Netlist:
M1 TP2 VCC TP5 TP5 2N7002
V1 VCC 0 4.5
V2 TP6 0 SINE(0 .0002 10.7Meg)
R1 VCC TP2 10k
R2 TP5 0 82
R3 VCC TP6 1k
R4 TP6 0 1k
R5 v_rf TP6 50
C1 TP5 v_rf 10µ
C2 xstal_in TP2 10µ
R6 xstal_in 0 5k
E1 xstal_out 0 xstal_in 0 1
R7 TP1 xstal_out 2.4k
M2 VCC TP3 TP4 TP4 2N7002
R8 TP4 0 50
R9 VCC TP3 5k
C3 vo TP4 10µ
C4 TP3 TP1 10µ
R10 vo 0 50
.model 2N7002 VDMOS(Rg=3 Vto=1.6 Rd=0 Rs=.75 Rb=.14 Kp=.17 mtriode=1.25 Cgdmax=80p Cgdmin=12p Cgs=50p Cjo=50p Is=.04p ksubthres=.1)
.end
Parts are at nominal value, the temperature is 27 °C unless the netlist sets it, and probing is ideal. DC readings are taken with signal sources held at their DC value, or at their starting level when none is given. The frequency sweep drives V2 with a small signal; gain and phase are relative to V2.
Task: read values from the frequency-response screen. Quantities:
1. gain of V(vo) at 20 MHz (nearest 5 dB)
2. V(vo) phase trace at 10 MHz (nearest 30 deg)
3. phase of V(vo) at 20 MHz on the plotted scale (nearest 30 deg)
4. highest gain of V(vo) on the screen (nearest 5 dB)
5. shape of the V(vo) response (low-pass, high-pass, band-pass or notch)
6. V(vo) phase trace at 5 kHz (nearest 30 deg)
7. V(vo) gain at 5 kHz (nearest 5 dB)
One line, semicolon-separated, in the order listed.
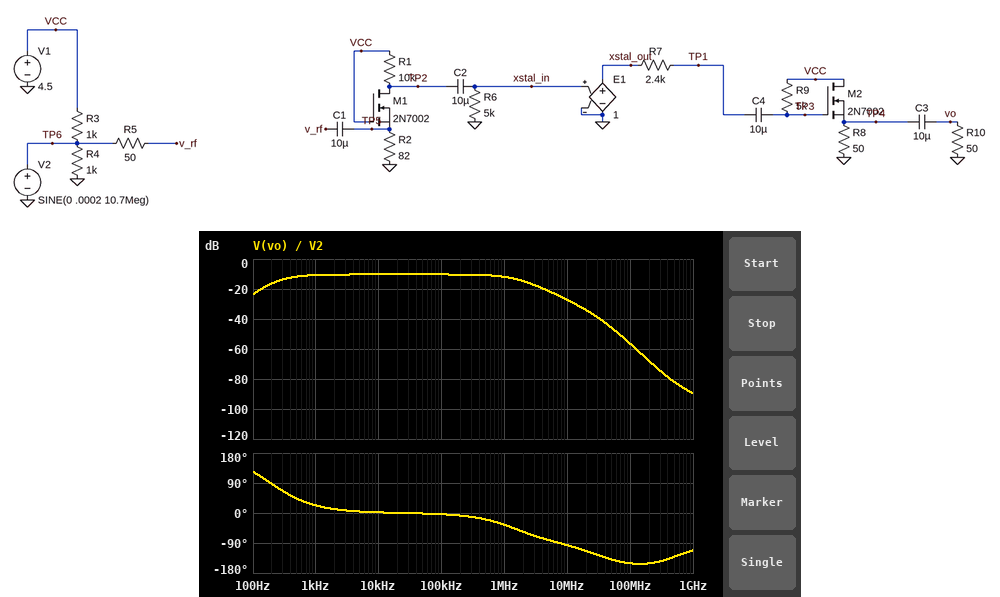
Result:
-35 dB; -90 deg; -120 deg; -10 dB; band-pass; 0 deg; -10 dB
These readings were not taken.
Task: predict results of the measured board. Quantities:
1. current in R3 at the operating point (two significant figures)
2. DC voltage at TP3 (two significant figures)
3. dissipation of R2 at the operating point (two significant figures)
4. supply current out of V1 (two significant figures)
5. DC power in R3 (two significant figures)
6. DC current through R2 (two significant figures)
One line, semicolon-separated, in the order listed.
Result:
4.5 mA; 4.5 V; 16 µW; 48 mA; 20 mW; 450 µA
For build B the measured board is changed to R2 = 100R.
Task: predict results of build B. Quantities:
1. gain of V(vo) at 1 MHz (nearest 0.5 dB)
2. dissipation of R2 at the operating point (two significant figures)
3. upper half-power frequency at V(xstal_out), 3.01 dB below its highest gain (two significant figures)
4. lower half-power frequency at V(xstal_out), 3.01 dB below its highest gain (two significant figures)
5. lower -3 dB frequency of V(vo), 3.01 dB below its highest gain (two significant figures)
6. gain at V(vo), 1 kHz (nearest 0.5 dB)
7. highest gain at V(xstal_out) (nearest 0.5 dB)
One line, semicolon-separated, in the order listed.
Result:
-11.5 dB; 20 µW; 33 MHz; 110 Hz; 310 Hz; -10.0 dB; -3.5 dB
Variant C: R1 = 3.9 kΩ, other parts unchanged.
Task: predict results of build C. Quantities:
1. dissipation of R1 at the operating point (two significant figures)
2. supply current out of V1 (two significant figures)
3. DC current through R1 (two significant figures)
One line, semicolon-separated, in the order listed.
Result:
5.0 mW; 49 mA; 1.1 mA
